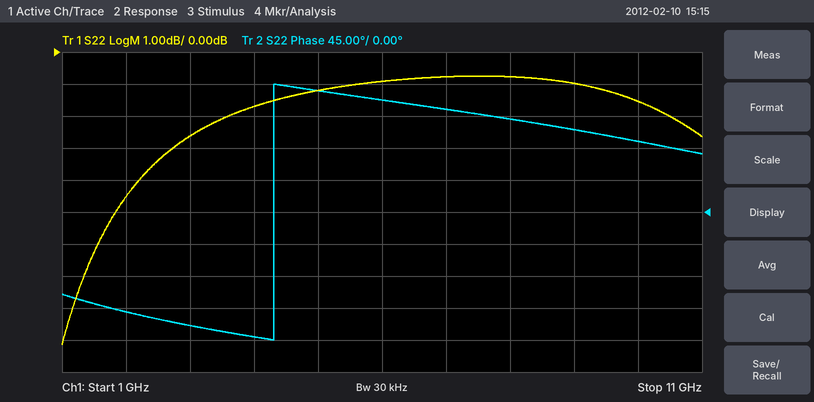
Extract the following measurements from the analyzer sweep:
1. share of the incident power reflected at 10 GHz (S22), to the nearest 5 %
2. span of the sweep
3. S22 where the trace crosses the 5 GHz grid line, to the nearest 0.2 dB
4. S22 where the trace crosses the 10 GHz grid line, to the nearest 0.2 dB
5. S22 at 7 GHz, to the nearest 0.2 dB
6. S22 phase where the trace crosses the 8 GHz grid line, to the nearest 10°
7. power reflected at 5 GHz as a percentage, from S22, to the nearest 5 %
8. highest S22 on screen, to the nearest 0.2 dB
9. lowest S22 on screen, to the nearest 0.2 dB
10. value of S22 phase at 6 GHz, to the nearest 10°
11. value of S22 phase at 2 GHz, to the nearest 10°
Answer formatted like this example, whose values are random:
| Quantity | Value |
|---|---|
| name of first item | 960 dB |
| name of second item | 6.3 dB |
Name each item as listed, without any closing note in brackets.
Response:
| Quantity | Value |
|---|---|
| share of the incident power reflected at 10 GHz (S22), to the nearest 5 % | 70 % |
| span of the sweep | 10 GHz |
| S22 where the trace crosses the 5 GHz grid line, to the nearest 0.2 dB | -1.2 dB |
| S22 where the trace crosses the 10 GHz grid line, to the nearest 0.2 dB | -1.6 dB |
| S22 at 7 GHz, to the nearest 0.2 dB | -0.8 dB |
| S22 phase where the trace crosses the 8 GHz grid line, to the nearest 10° | 130° |
| power reflected at 5 GHz as a percentage, from S22, to the nearest 5 % | 75 % |
| highest S22 on screen, to the nearest 0.2 dB | -0.8 dB |
| lowest S22 on screen, to the nearest 0.2 dB | -9.2 dB |
| value of S22 phase at 6 GHz, to the nearest 10° | 160° |
| value of S22 phase at 2 GHz, to the nearest 10° | -140° |
